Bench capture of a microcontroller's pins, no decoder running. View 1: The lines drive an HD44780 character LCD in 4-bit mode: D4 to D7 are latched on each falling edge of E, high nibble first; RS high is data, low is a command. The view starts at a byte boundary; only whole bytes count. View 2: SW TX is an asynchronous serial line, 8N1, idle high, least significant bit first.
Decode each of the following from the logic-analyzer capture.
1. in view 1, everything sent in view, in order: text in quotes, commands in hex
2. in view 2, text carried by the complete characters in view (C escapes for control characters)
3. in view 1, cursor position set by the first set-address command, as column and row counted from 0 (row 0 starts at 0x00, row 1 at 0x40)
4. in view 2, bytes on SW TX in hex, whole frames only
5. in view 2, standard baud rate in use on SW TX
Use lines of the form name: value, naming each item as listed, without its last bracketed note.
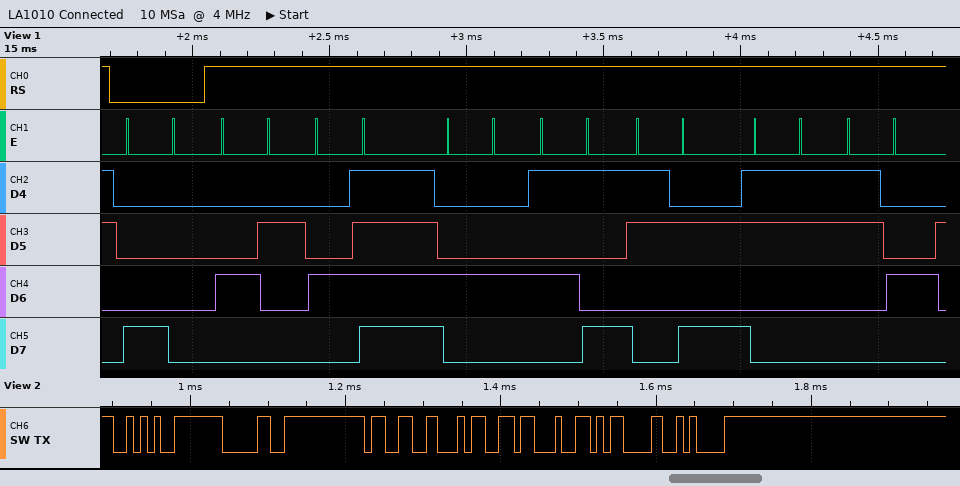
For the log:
in view 1, everything sent in view, in order: text in quotes, commands in hex: 0x80 "BODY:34"
in view 2, text carried by the complete characters in view: "*034#\r\n"
in view 1, cursor position set by the first set-address command, as column and row counted from 0: column 0, row 0
in view 2, bytes on SW TX in hex, whole frames only: 2A 30 33 34 23 0D 0A
in view 2, standard baud rate in use on SW TX: 115200 baud
